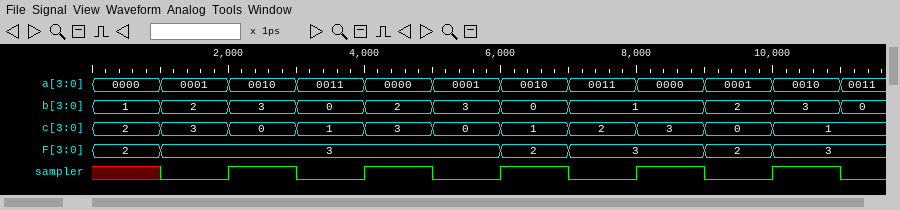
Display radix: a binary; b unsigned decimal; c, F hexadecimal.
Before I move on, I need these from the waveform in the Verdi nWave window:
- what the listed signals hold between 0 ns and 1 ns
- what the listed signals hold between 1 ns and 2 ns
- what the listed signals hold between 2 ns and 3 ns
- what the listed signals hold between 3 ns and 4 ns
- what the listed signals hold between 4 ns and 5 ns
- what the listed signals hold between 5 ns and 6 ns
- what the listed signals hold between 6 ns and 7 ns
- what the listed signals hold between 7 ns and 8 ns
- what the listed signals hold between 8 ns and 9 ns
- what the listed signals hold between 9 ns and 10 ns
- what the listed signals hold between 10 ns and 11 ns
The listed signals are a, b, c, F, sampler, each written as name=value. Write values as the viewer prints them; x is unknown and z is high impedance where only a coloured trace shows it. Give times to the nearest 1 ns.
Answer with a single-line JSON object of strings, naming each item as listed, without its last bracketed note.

{"what the listed signals hold between 0 ns and 1 ns": "a=0000, b=1, c=2, F=2, sampler=x", "what the listed signals hold between 1 ns and 2 ns": "a=0001, b=2, c=3, F=3, sampler=0", "what the listed signals hold between 2 ns and 3 ns": "a=0010, b=3, c=0, F=3, sampler=1", "what the listed signals hold between 3 ns and 4 ns": "a=0011, b=0, c=1, F=3, sampler=0", "what the listed signals hold between 4 ns and 5 ns": "a=0000, b=2, c=3, F=3, sampler=1", "what the listed signals hold between 5 ns and 6 ns": "a=0001, b=3, c=0, F=3, sampler=0", "what the listed signals hold between 6 ns and 7 ns": "a=0010, b=0, c=1, F=2, sampler=1", "what the listed signals hold between 7 ns and 8 ns": "a=0011, b=1, c=2, F=3, sampler=0", "what the listed signals hold between 8 ns and 9 ns": "a=0000, b=1, c=3, F=3, sampler=1", "what the listed signals hold between 9 ns and 10 ns": "a=0001, b=2, c=0, F=2, sampler=0", "what the listed signals hold between 10 ns and 11 ns": "a=0010, b=3, c=1, F=3, sampler=1"}
